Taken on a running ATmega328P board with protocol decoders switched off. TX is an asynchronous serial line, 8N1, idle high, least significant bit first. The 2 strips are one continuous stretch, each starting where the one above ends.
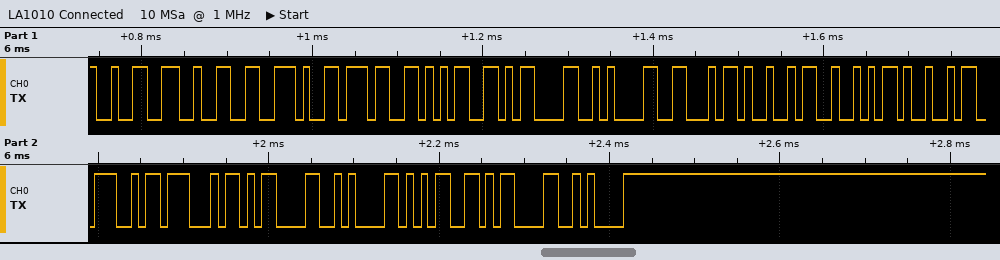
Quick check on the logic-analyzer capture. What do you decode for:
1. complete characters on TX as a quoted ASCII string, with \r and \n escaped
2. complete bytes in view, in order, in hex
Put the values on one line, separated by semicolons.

"22.75\r\nFIRING\r\n5\r\n"; 32 32 2E 37 35 0D 0A 46 49 52 49 4E 47 0D 0A 35 0D 0A
